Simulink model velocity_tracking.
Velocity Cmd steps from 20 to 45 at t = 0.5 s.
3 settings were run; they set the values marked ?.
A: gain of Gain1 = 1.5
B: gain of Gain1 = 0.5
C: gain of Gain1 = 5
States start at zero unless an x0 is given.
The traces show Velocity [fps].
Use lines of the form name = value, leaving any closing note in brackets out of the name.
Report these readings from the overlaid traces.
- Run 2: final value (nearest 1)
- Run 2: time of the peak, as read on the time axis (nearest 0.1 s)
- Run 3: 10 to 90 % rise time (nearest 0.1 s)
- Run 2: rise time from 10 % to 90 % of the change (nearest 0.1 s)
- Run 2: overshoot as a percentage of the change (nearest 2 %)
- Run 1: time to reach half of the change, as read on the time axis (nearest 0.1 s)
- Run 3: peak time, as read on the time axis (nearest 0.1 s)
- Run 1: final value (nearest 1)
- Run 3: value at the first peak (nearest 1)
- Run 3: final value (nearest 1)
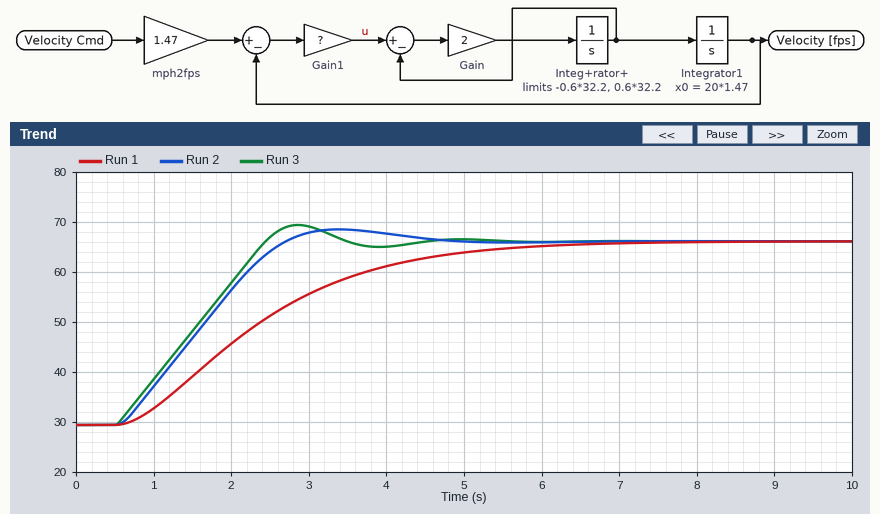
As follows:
Run 2: final value = 66
Run 2: time of the peak, as read on the time axis = 3.4 s
Run 3: 10 to 90 % rise time = 1.5 s
Run 2: rise time from 10 % to 90 % of the change = 1.6 s
Run 2: overshoot as a percentage of the change = 6 %
Run 1: time to reach half of the change, as read on the time axis = 2.2 s
Run 3: peak time, as read on the time axis = 2.9 s
Run 1: final value = 66
Run 3: value at the first peak = 69
Run 3: final value = 66
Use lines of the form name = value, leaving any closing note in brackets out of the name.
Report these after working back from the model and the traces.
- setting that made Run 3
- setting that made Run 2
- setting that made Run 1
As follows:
setting that made Run 3 = C
setting that made Run 2 = A
setting that made Run 1 = B
